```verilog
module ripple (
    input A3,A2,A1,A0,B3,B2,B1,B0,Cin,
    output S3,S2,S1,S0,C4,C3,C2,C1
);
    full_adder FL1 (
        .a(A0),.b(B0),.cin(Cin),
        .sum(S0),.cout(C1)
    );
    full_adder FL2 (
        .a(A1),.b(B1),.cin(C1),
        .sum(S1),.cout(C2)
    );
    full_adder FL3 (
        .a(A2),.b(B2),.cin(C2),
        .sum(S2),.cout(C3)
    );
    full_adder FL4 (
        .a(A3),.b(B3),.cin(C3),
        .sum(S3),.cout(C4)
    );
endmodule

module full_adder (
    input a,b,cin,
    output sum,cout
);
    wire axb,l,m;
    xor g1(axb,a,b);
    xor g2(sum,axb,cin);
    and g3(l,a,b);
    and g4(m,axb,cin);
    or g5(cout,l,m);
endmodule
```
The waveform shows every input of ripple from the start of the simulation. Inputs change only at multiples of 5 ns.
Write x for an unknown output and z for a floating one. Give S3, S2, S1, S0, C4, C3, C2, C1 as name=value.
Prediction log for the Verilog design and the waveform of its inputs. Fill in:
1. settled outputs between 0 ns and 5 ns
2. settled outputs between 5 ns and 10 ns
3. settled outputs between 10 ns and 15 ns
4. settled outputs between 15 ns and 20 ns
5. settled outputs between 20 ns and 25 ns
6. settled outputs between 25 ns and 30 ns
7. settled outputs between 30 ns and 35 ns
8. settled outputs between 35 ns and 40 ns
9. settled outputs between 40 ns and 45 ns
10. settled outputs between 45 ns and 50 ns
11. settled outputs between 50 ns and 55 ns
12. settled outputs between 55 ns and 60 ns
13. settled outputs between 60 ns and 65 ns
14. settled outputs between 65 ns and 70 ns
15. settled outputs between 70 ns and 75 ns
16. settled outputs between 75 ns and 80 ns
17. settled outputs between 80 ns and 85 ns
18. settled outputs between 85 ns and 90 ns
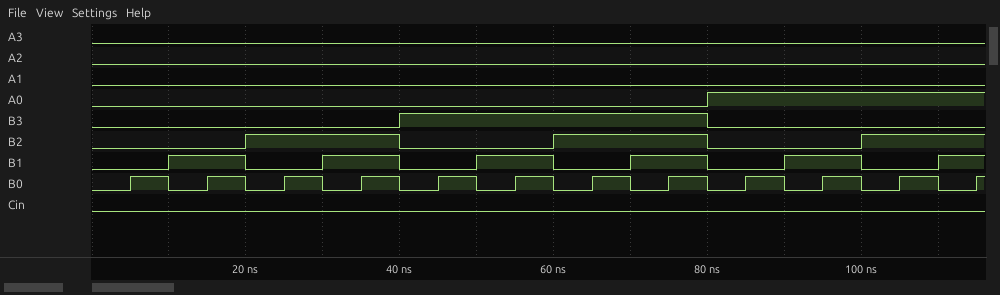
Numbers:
S3=0, S2=0, S1=0, S0=0, C4=0, C3=0, C2=0, C1=0
S3=0, S2=0, S1=0, S0=1, C4=0, C3=0, C2=0, C1=0
S3=0, S2=0, S1=1, S0=0, C4=0, C3=0, C2=0, C1=0
S3=0, S2=0, S1=1, S0=1, C4=0, C3=0, C2=0, C1=0
S3=0, S2=1, S1=0, S0=0, C4=0, C3=0, C2=0, C1=0
S3=0, S2=1, S1=0, S0=1, C4=0, C3=0, C2=0, C1=0
S3=0, S2=1, S1=1, S0=0, C4=0, C3=0, C2=0, C1=0
S3=0, S2=1, S1=1, S0=1, C4=0, C3=0, C2=0, C1=0
S3=1, S2=0, S1=0, S0=0, C4=0, C3=0, C2=0, C1=0
S3=1, S2=0, S1=0, S0=1, C4=0, C3=0, C2=0, C1=0
S3=1, S2=0, S1=1, S0=0, C4=0, C3=0, C2=0, C1=0
S3=1, S2=0, S1=1, S0=1, C4=0, C3=0, C2=0, C1=0
S3=1, S2=1, S1=0, S0=0, C4=0, C3=0, C2=0, C1=0
S3=1, S2=1, S1=0, S0=1, C4=0, C3=0, C2=0, C1=0
S3=1, S2=1, S1=1, S0=0, C4=0, C3=0, C2=0, C1=0
S3=1, S2=1, S1=1, S0=1, C4=0, C3=0, C2=0, C1=0
S3=0, S2=0, S1=0, S0=1, C4=0, C3=0, C2=0, C1=0
S3=0, S2=0, S1=1, S0=0, C4=0, C3=0, C2=0, C1=1
